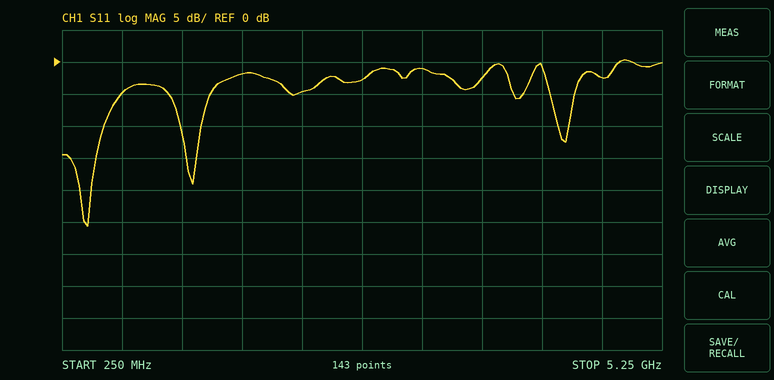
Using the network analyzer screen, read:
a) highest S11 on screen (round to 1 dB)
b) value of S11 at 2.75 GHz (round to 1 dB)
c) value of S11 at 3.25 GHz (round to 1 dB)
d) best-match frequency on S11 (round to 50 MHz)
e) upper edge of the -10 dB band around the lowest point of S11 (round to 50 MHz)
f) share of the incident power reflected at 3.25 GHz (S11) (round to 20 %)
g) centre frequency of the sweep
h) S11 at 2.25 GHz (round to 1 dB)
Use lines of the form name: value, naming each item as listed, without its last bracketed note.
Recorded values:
highest S11 on screen: 0 dB
value of S11 at 2.75 GHz: -3 dB
value of S11 at 3.25 GHz: -1 dB
best-match frequency on S11: 450 MHz
upper edge of the -10 dB band around the lowest point of S11: 600 MHz
share of the incident power reflected at 3.25 GHz (S11): 80 %
centre frequency of the sweep: 2.75 GHz
S11 at 2.25 GHz: -5 dB
